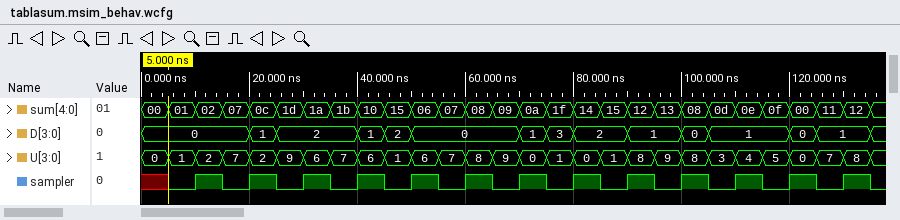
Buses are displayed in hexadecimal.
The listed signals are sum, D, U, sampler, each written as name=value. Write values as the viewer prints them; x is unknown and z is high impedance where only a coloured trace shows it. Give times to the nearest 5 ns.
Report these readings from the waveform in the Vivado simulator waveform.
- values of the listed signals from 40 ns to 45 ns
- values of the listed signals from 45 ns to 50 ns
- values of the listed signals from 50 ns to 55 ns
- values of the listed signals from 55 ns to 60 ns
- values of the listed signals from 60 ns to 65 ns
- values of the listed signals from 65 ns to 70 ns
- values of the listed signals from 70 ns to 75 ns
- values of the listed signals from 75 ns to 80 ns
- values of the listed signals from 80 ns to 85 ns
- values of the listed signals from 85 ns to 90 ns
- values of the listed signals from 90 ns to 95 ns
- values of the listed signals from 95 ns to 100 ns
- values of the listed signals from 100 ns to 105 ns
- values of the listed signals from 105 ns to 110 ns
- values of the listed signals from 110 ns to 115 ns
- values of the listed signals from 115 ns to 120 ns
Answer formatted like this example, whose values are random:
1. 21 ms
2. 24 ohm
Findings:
1. sum=10, D=1, U=6, sampler=1
2. sum=15, D=2, U=1, sampler=0
3. sum=06, D=0, U=6, sampler=1
4. sum=07, D=0, U=7, sampler=0
5. sum=08, D=0, U=8, sampler=1
6. sum=09, D=0, U=9, sampler=0
7. sum=0a, D=1, U=0, sampler=1
8. sum=1f, D=3, U=1, sampler=0
9. sum=14, D=2, U=0, sampler=1
10. sum=15, D=2, U=1, sampler=0
11. sum=12, D=1, U=8, sampler=1
12. sum=13, D=1, U=9, sampler=0
13. sum=08, D=0, U=8, sampler=1
14. sum=0d, D=1, U=3, sampler=0
15. sum=0e, D=1, U=4, sampler=1
16. sum=0f, D=1, U=5, sampler=0
